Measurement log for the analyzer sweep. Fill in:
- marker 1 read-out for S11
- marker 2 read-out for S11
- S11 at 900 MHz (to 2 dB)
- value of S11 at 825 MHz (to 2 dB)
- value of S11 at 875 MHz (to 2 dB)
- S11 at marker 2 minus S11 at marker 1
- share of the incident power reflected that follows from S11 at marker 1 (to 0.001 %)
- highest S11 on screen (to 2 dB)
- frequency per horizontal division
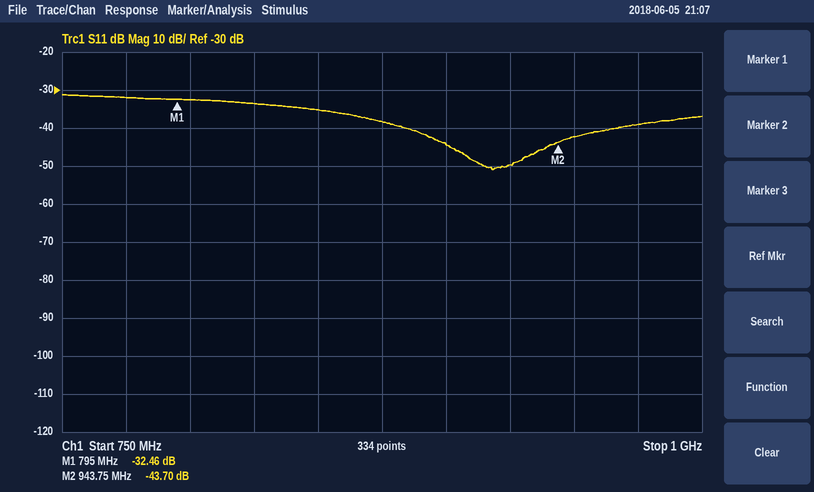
-32.46 dB
-43.70 dB
-44 dB
-34 dB
-38 dB
-11.24 dB
0.057 %
-32 dB
25 MHz
